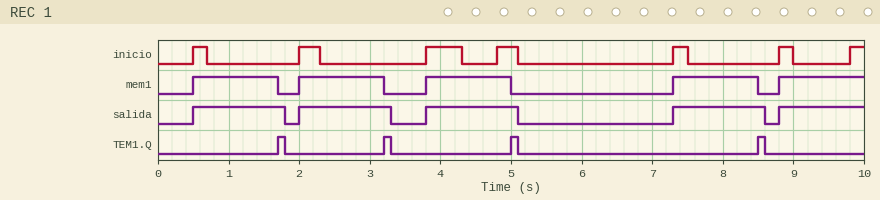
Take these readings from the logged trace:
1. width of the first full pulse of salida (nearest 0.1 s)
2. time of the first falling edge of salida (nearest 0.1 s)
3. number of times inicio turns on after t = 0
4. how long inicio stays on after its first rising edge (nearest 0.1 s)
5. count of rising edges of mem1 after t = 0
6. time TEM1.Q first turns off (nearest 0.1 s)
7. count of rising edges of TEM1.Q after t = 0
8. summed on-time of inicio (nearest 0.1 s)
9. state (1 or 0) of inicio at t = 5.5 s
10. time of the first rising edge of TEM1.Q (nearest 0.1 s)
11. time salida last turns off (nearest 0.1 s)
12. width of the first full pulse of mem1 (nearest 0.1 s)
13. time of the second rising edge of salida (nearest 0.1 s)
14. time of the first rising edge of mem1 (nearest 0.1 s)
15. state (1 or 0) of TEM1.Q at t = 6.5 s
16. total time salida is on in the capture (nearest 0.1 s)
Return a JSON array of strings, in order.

["1.3 s", "1.8 s", "7", "0.2 s", "5", "1.8 s", "4", "1.9 s", "0", "1.7 s", "8.6 s", "1.2 s", "2.0 s", "0.5 s", "0", "6.4 s"]
